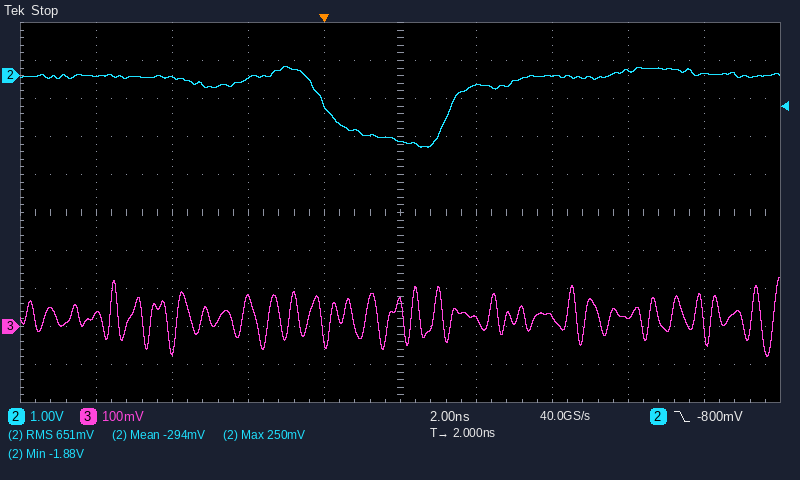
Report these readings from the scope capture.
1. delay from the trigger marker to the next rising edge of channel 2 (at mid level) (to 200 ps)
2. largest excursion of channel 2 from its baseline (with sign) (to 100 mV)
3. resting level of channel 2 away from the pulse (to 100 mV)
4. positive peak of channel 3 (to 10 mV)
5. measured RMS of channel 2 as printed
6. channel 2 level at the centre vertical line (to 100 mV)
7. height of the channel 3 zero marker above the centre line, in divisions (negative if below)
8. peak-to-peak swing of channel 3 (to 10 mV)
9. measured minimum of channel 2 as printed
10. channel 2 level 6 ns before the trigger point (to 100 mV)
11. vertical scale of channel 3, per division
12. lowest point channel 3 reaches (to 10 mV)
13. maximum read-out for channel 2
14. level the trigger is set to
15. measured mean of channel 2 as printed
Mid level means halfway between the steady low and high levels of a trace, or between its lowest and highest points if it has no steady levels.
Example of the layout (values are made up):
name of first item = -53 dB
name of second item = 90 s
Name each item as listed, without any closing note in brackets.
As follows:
delay from the trigger marker to the next rising edge of channel 2 (at mid level) = 3.4 ns
largest excursion of channel 2 from its baseline (with sign) = -1.9 V
resting level of channel 2 away from the pulse = 0.0 V
positive peak of channel 3 = 130 mV
measured RMS of channel 2 as printed = 651 mV
channel 2 level at the centre vertical line = -1.7 V
height of the channel 3 zero marker above the centre line, in divisions = -3.0 div
peak-to-peak swing of channel 3 = 210 mV
measured minimum of channel 2 as printed = -1.88 V
channel 2 level 6 ns before the trigger point = 0.0 V
vertical scale of channel 3, per division = 100 mV
lowest point channel 3 reaches = -80 mV
maximum read-out for channel 2 = 250 mV
level the trigger is set to = -800 mV
measured mean of channel 2 as printed = -294 mV
